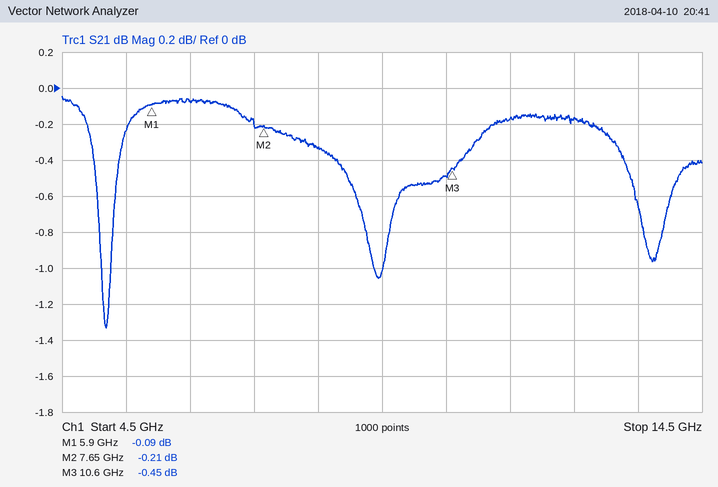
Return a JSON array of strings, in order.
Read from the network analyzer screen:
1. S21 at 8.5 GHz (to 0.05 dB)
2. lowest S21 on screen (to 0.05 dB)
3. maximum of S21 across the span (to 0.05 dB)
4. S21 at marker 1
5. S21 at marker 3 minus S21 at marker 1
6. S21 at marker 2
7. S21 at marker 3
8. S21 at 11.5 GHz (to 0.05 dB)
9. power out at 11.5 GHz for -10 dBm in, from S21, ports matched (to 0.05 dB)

["-0.35 dB", "-1.35 dB", "-0.05 dB", "-0.09 dB", "-0.36 dB", "-0.21 dB", "-0.45 dB", "-0.15 dB", "-10.15 dBm"]
